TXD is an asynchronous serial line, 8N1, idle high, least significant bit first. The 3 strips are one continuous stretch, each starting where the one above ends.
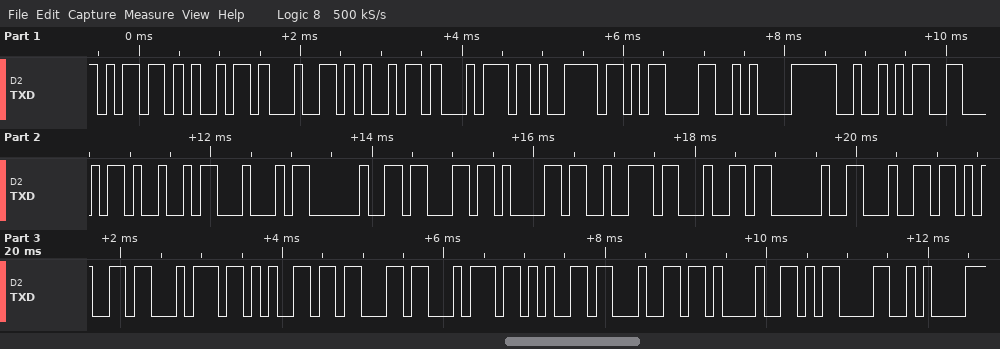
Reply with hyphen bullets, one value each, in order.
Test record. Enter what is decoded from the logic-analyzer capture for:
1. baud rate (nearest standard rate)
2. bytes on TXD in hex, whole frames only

- 9600 baud
- 6D 69 64 69 74 79 0D 0A 52 46 49 44 20 63 61 72 64 20 64 65 74 65 63 74 65 64 21 0D 0A
